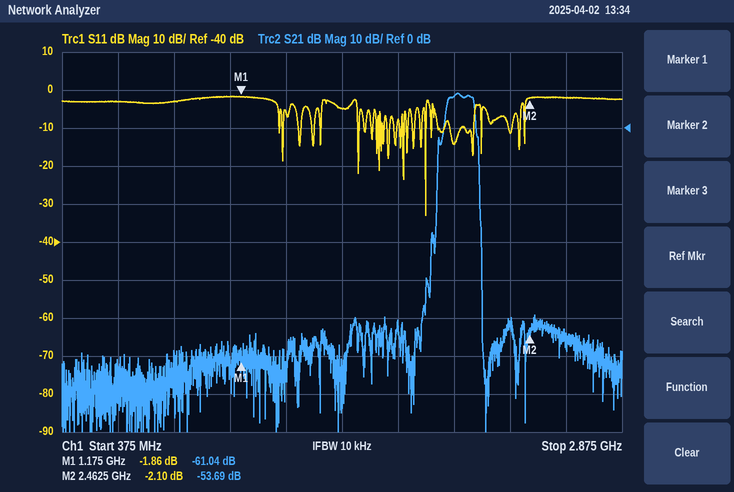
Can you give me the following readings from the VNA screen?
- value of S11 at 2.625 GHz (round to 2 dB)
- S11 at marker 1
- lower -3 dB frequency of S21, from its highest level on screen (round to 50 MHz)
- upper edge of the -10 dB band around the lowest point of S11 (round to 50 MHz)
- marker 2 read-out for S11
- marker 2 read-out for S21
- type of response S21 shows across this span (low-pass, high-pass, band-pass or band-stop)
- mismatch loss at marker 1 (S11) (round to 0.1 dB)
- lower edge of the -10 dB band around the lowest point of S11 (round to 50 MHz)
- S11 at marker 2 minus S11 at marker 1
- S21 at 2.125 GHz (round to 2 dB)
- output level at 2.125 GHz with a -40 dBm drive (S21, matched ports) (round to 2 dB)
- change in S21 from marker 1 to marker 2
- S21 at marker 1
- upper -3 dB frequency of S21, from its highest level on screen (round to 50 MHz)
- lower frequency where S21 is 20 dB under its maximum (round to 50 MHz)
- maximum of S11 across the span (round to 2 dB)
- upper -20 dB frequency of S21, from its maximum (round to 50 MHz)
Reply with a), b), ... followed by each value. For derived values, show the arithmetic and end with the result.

a) -2 dB
b) -1.86 dB
c) 2.10 GHz
d) 2.00 GHz
e) -2.10 dB
f) -53.69 dB
g) band-pass
h) −10 log10(1 − 10^(-1.86/10)) ≈ 4.6 dB
i) 2.00 GHz
j) -2.1 − (-1.86) = -0.24 dB
k) 8 dB
l) -40 dBm + (8 dB) = -32 dBm
m) -53.69 − (-61.04) = 7.35 dB
n) -61.04 dB
o) 2.20 GHz
p) 2.05 GHz
q) -2 dB
r) 2.25 GHz
